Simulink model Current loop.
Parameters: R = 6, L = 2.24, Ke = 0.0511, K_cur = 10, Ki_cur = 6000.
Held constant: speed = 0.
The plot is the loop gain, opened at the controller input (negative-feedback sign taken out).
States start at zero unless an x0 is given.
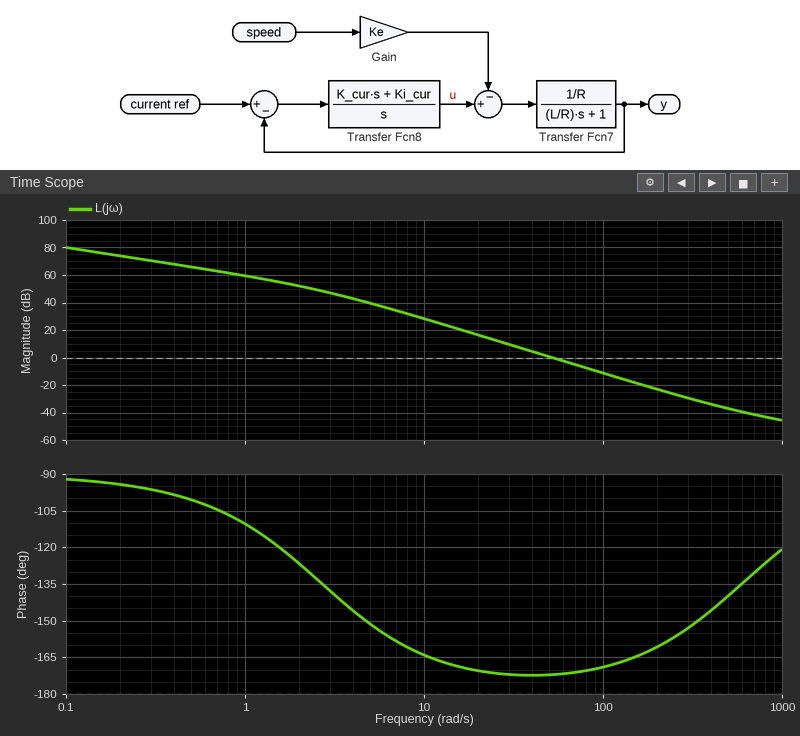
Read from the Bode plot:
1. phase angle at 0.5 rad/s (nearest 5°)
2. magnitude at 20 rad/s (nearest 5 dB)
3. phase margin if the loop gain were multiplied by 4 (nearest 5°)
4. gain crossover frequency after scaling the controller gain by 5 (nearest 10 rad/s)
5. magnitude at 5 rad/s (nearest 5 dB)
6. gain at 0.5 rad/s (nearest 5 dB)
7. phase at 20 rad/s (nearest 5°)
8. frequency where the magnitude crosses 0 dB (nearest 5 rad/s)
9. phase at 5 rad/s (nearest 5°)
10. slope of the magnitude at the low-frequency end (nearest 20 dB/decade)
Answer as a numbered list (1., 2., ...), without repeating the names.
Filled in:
1. -100°
2. 15 dB
3. 10°
4. 120 rad/s
5. 40 dB
6. 65 dB
7. -170°
8. 50 rad/s
9. -150°
10. -20 dB/decade
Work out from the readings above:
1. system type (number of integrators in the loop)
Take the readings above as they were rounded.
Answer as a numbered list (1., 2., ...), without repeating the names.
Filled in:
1. 1
